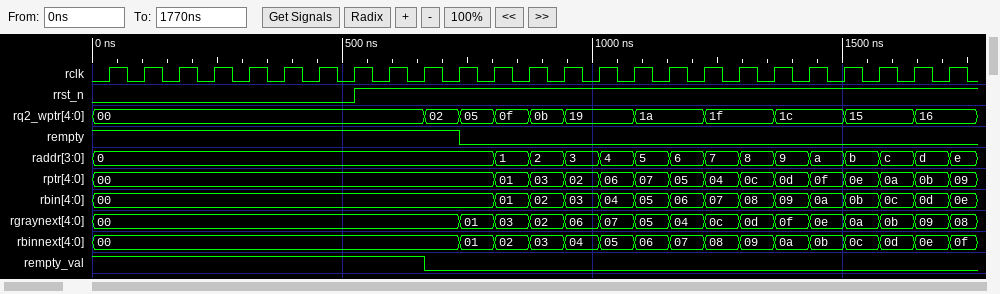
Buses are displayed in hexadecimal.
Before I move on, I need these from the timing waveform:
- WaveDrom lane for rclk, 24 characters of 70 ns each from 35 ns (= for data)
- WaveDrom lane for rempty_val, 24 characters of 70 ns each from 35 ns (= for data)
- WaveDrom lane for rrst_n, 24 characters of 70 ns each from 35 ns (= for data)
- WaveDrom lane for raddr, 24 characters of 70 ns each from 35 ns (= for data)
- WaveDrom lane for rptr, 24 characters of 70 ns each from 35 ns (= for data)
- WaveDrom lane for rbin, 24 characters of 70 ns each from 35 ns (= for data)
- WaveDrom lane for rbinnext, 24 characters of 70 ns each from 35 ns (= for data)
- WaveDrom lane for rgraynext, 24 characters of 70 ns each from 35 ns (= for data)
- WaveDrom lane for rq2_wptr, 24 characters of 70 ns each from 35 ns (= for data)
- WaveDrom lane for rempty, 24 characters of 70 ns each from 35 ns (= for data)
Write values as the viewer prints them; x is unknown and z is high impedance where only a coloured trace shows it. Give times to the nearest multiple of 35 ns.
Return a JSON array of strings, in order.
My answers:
["{name: 'rclk', wave: 'p.......................'}", "{name: 'rempty_val', wave: '1........0..............'}", "{name: 'rrst_n', wave: '0......1................'}", "{name: 'raddr', wave: '=..........=============', data: '0 1 2 3 4 5 6 7 8 9 a b c d'}", "{name: 'rptr', wave: '=..........=============', data: '00 01 03 02 06 07 05 04 0c 0d 0f 0e 0a 0b'}", "{name: 'rbin', wave: '=..........=============', data: '00 01 02 03 04 05 06 07 08 09 0a 0b 0c 0d'}", "{name: 'rbinnext', wave: '=.........==============', data: '00 01 02 03 04 05 06 07 08 09 0a 0b 0c 0d 0e'}", "{name: 'rgraynext', wave: '=.........==============', data: '00 01 03 02 06 07 05 04 0c 0d 0f 0e 0a 0b 09'}", "{name: 'rq2_wptr', wave: '=........=====.=.=.=.=.=', data: '00 02 05 0f 0b 19 1a 1f 1c 15 16'}", "{name: 'rempty', wave: '1.........0.............'}"]
